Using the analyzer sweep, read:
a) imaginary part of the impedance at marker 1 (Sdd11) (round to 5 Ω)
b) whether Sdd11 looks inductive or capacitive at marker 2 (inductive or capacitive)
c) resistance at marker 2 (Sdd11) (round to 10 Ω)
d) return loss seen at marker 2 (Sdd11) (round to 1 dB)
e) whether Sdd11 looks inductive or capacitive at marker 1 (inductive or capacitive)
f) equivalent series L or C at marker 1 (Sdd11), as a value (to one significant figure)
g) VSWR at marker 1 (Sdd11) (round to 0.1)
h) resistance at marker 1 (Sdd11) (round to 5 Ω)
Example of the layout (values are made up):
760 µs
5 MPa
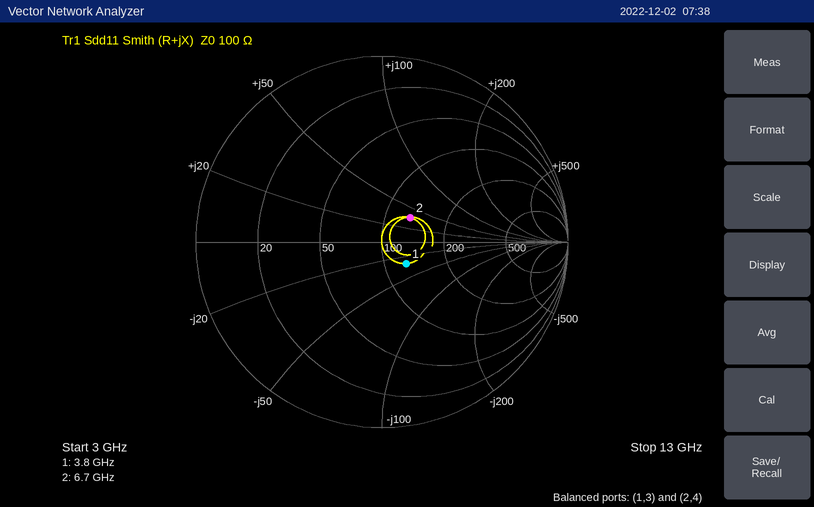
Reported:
-30 Ω
inductive
130 Ω
14 dB
capacitive
1 pF
1.4
125 Ω
